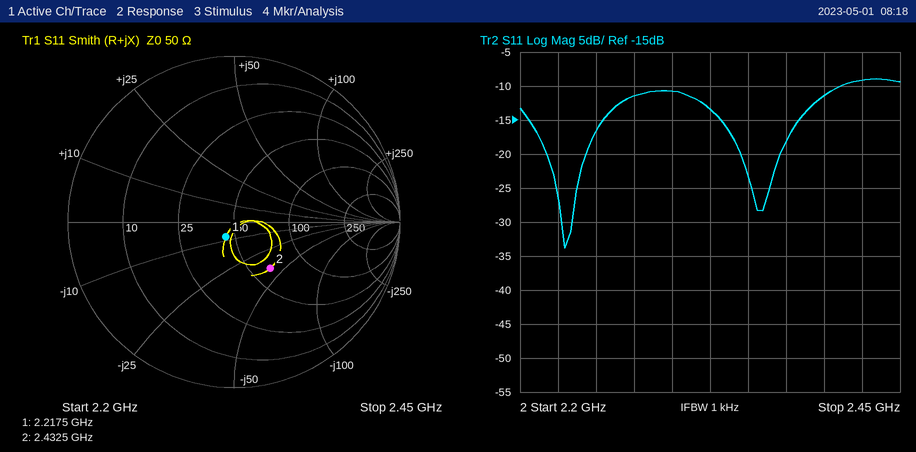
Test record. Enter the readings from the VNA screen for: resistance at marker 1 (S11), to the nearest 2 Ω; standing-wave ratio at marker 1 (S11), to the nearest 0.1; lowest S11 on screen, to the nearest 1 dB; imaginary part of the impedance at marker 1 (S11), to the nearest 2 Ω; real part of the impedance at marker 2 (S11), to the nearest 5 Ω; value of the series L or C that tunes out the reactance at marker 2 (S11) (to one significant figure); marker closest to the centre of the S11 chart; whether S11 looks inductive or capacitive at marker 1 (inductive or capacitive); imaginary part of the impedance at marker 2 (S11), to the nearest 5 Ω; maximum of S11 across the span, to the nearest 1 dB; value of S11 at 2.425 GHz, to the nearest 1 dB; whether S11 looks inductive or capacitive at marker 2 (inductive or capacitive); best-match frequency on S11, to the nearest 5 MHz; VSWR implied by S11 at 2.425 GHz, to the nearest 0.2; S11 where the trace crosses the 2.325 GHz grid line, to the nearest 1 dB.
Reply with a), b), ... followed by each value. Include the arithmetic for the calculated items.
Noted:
a) 44 Ω
b) 1.2
c) -34 dB
d) -8 Ω
e) 65 Ω
f) L = 40 Ω/(2π × 2.4325 GHz) ≈ 3 nH
g) marker 1
h) capacitive
i) -40 Ω
j) -9 dB
k) -9 dB
l) capacitive
m) 2.230 GHz
n) |Γ| = 10^(-9/20) = 0.3548; VSWR = (1 + 0.3548)/(1 − 0.3548) ≈ 2.10, so 2.0 to the nearest 0.2
o) -13 dB
